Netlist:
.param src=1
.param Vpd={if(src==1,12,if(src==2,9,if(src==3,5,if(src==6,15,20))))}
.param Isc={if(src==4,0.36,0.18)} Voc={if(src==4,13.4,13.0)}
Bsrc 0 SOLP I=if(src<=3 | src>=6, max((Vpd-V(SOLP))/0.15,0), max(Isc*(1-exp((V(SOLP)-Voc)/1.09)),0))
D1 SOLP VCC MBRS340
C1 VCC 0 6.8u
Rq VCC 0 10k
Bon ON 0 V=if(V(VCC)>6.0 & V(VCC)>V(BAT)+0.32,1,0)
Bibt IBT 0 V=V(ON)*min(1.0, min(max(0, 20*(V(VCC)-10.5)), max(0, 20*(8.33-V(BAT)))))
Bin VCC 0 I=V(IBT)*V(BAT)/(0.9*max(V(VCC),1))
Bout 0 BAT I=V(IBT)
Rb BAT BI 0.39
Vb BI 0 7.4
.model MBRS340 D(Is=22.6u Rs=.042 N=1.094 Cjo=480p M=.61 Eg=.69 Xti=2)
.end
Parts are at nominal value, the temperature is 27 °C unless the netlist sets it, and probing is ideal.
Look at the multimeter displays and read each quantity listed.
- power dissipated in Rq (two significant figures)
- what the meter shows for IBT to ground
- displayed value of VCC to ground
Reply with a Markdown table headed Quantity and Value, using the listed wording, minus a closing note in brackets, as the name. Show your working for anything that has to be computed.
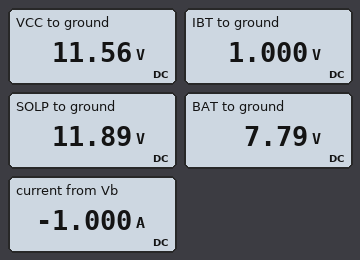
| Quantity | Value |
|---|---|
| power dissipated in Rq | (11.56 V)^2 / 10 kΩ = 13 mW |
| what the meter shows for IBT to ground | 1.000 V |
| displayed value of VCC to ground | 11.56 V |
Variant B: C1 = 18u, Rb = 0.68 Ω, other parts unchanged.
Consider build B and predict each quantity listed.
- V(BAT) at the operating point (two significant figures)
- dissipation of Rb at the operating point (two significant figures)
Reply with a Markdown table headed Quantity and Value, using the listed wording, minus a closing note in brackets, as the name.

| Quantity | Value |
|---|---|
| V(BAT) at the operating point | 8.1 V |
| dissipation of Rb at the operating point | 680 mW |
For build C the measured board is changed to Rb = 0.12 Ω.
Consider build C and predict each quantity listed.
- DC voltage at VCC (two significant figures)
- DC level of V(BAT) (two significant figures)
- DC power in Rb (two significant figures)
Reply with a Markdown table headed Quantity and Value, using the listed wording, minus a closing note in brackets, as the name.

| Quantity | Value |
|---|---|
| DC voltage at VCC | 12 V |
| DC level of V(BAT) | 7.5 V |
| DC power in Rb | 120 mW |
